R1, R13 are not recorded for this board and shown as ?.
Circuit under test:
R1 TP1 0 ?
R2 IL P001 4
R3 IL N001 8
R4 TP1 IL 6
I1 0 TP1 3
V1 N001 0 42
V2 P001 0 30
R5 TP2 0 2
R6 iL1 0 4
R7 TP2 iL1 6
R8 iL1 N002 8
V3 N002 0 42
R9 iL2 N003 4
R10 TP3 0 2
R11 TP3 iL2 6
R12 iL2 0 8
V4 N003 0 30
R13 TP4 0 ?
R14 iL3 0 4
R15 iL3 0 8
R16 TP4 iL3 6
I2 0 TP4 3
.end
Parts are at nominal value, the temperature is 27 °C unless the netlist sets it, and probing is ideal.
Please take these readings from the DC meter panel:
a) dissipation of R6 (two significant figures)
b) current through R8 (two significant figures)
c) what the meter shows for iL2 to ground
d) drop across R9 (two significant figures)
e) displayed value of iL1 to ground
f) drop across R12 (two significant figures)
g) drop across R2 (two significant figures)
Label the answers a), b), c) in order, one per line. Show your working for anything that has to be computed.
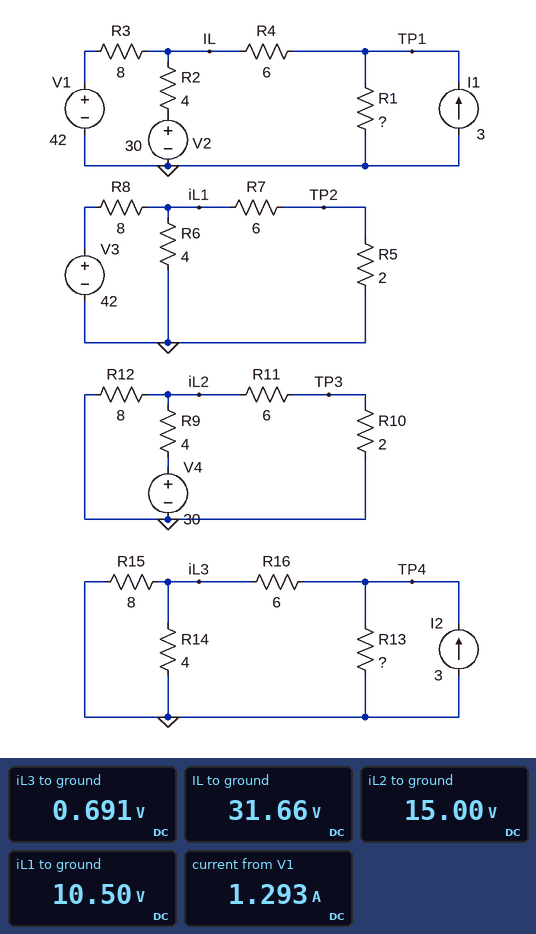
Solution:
a) (10.5 V)^2 / 4 Ω = 28 W
b) (42 V - 10.5 V) / 8 Ω = 3.9 A
c) 15.00 V
d) 30 V - 15 V = 15 V
e) 10.50 V
f) 15 V = 15 V
g) 31.66 V - 30 V = 1.7 V
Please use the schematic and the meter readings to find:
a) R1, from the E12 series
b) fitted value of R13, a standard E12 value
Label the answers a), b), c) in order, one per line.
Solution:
a) 6.8 Ω
b) 0.82 Ω
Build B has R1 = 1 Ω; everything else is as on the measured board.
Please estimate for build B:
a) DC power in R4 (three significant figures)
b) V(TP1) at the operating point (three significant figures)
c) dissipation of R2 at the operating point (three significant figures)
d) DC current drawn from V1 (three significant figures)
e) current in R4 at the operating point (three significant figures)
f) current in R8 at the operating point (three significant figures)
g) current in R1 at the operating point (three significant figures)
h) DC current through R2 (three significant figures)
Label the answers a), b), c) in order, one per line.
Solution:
a) 61.7 W
b) 6.21 V
c) 5.18 W
d) 2.07 A
e) 3.21 A
f) 3.94 A
g) 6.21 A
h) 1.14 A
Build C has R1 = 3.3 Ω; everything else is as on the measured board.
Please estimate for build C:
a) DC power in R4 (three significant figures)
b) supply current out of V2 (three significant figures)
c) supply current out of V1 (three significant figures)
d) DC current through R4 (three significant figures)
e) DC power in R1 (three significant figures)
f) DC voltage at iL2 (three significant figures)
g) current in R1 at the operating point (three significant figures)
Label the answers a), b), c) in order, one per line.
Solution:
a) 24.3 W
b) 343 mA
c) 1.67 A
d) 2.01 A
e) 83.0 W
f) 15.0 V
g) 5.01 A
